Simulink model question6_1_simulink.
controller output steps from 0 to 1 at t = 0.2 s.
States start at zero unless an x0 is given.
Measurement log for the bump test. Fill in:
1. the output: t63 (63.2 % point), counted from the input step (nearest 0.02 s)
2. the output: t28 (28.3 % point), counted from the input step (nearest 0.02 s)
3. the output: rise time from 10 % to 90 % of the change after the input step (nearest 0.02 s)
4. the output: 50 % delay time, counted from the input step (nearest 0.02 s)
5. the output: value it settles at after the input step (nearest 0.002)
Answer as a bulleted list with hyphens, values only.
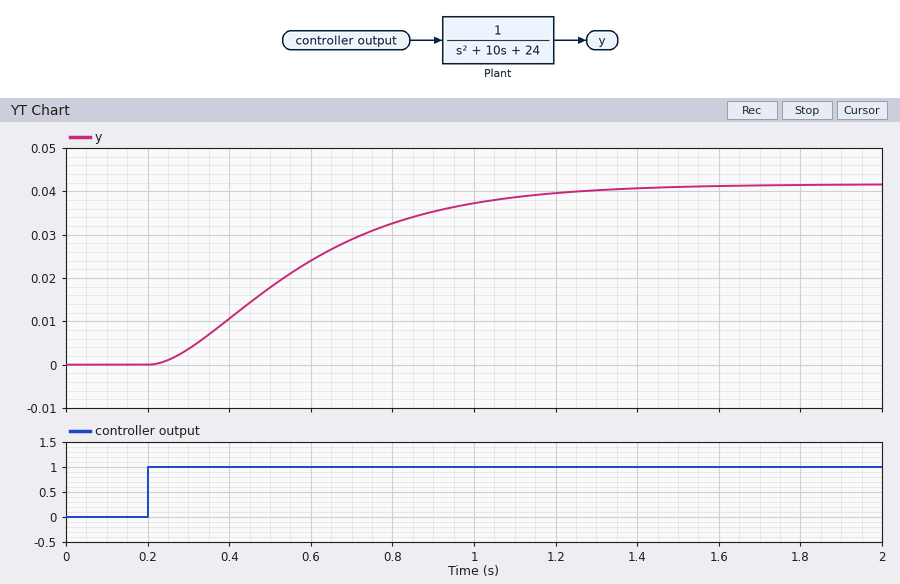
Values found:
- 0.44 s
- 0.22 s
- 0.70 s
- 0.34 s
- 0.042
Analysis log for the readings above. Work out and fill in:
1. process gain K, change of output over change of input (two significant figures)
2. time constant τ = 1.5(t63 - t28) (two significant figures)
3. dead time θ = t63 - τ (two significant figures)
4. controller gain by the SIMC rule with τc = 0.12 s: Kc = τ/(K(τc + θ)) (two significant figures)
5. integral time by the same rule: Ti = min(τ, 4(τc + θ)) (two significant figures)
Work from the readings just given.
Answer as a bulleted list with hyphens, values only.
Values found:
- 0.042
- 0.33 s
- 0.11 s
- 34
- 0.33 s
